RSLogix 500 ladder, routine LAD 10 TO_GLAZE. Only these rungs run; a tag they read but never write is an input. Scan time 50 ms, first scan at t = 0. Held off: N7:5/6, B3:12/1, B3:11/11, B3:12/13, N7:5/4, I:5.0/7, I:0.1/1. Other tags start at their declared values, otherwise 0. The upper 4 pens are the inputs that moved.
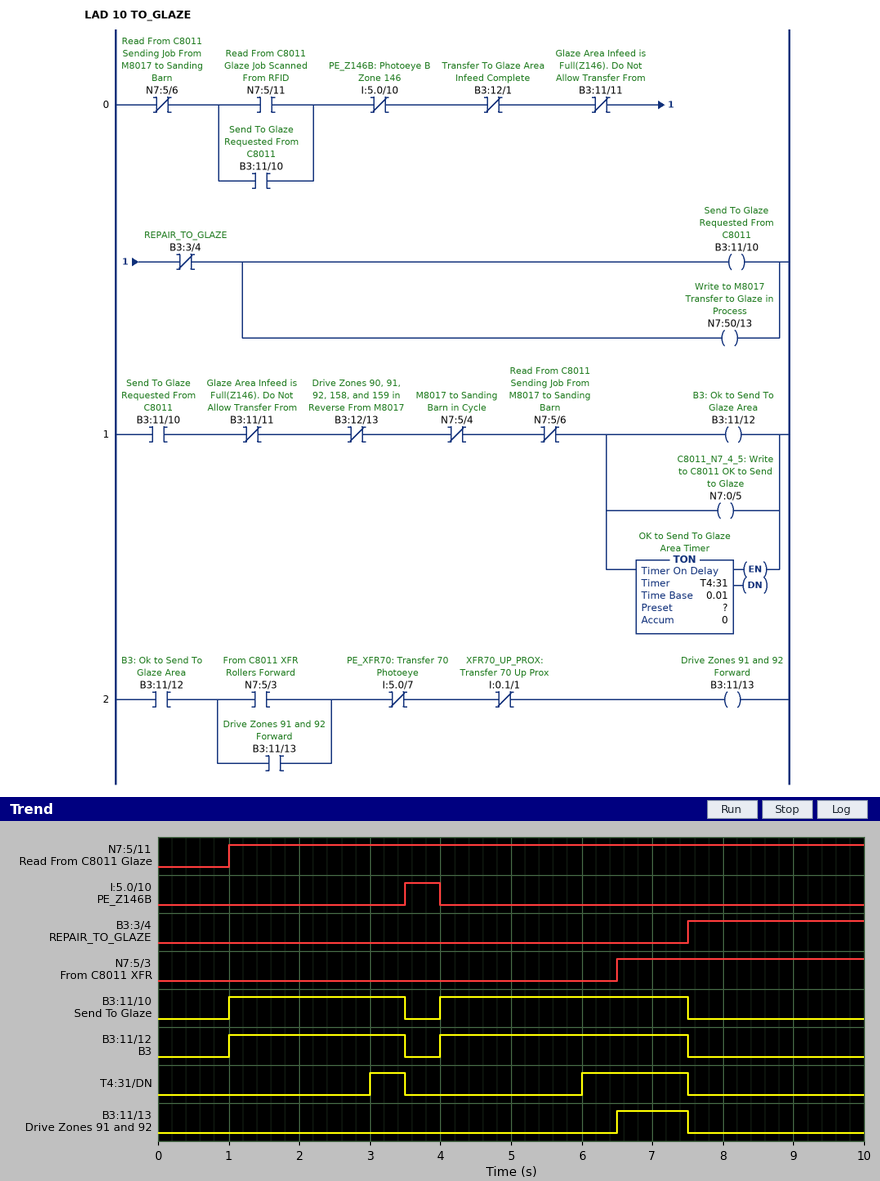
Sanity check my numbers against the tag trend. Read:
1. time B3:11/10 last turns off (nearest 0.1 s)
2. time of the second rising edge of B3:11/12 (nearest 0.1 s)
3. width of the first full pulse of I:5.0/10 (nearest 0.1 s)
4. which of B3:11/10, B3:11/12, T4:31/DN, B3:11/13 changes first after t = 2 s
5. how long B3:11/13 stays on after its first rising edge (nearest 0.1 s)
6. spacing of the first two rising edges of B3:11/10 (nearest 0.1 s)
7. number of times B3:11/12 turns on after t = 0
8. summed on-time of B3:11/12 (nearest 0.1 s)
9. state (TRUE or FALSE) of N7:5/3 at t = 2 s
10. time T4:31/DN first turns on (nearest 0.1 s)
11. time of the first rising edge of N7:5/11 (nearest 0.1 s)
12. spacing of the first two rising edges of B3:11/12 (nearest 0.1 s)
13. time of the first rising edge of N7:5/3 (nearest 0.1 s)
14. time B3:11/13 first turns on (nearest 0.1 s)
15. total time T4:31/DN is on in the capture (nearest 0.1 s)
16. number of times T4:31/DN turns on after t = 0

7.5 s
4.0 s
0.5 s
T4:31/DN
1.0 s
3.0 s
2
6.0 s
FALSE
3.0 s
1.0 s
3.0 s
6.5 s
6.5 s
2.0 s
2
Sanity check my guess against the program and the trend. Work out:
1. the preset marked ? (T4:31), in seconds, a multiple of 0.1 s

2.0 s
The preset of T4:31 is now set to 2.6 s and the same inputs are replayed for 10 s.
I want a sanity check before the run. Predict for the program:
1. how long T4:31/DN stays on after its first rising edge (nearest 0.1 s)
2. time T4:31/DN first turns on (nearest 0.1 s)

0.9 s
6.6 s
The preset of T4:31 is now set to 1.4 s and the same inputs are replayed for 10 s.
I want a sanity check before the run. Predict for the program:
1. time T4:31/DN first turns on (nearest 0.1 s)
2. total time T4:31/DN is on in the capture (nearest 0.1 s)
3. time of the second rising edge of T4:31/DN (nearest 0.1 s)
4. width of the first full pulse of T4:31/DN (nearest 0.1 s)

2.4 s
3.2 s
5.4 s
1.1 s
